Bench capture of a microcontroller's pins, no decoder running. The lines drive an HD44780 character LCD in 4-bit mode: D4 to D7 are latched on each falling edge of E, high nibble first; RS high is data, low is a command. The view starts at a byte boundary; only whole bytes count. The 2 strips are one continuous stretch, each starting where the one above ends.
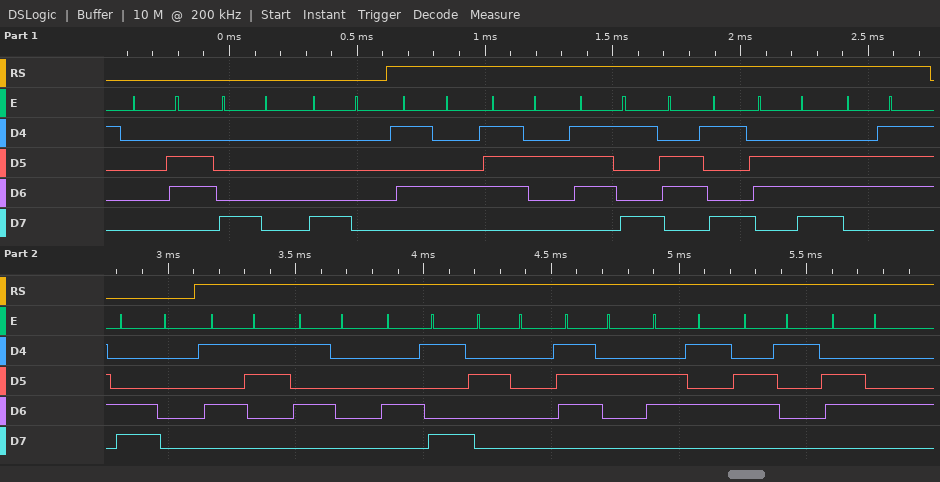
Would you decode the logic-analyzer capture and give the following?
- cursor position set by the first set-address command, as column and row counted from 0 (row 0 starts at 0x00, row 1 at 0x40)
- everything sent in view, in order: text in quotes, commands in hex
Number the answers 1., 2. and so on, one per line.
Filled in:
1. column 0, row 0
2. 0x06 0x80 0x80 "Trying" 0xC0 "SPI read"
